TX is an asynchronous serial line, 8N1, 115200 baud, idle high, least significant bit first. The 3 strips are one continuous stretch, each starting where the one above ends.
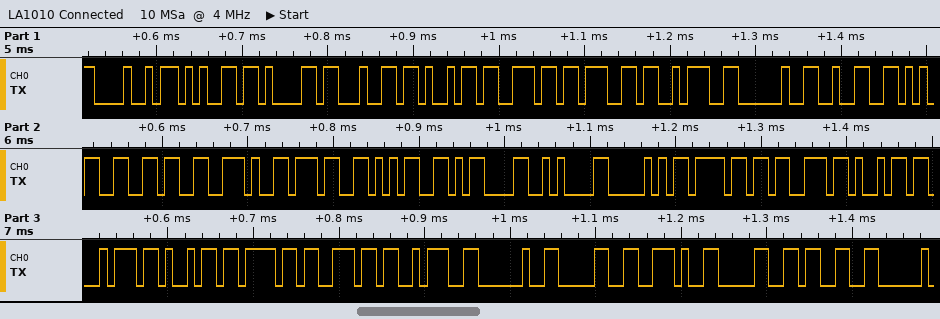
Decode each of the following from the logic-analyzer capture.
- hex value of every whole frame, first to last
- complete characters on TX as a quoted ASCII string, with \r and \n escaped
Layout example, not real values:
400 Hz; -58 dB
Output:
48 65 61 64 69 6E 67 3A 20 32 35 36 2E 37 35 0D 0A 50 6F 73 69 74 69 6F 6E 3A 20 30 2E 30 33; "Heading: 256.75\r\nPosition: 0.03"
